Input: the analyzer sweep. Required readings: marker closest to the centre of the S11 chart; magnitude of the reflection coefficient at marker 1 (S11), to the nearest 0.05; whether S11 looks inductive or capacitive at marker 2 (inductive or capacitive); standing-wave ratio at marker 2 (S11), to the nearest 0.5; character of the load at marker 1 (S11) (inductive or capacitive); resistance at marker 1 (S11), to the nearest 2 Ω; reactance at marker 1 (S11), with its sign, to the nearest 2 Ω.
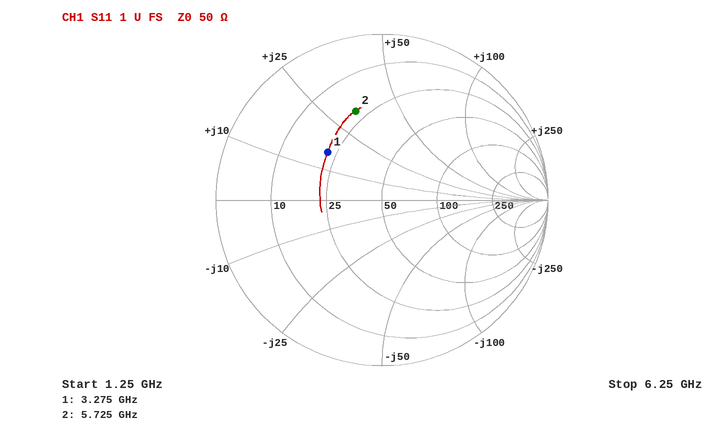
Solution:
marker 1
0.45
inductive
3.5
inductive
22 Ω
+16 Ω
